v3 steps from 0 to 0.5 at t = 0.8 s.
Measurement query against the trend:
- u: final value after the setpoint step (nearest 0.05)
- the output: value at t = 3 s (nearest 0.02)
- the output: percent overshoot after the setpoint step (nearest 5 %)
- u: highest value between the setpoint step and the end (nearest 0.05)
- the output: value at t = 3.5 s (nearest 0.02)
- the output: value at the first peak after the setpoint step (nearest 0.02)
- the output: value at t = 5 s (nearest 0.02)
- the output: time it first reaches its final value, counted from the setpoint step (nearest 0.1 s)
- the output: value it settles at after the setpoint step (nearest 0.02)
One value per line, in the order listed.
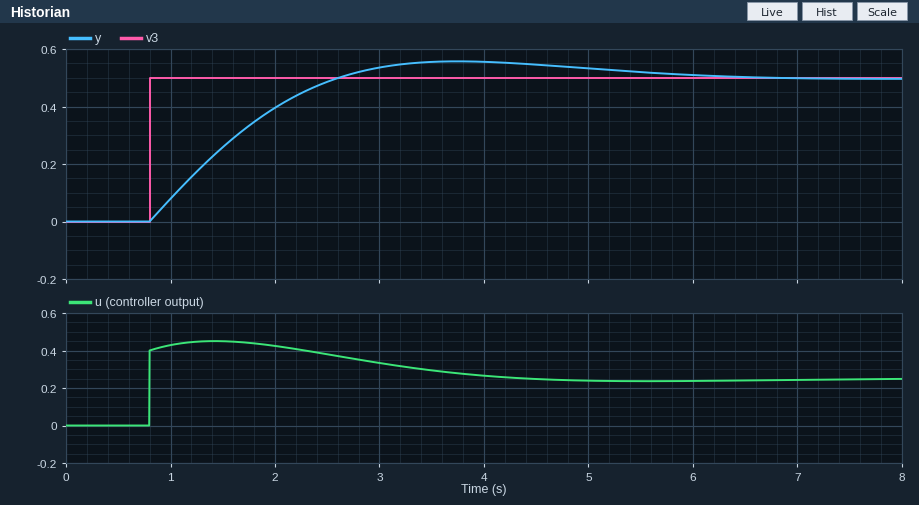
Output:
0.25
0.54
10 %
0.45
0.56
0.56
0.54
1.8 s
0.50
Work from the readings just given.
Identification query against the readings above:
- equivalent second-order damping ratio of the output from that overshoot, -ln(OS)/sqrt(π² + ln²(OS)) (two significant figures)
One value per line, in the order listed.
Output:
0.59
